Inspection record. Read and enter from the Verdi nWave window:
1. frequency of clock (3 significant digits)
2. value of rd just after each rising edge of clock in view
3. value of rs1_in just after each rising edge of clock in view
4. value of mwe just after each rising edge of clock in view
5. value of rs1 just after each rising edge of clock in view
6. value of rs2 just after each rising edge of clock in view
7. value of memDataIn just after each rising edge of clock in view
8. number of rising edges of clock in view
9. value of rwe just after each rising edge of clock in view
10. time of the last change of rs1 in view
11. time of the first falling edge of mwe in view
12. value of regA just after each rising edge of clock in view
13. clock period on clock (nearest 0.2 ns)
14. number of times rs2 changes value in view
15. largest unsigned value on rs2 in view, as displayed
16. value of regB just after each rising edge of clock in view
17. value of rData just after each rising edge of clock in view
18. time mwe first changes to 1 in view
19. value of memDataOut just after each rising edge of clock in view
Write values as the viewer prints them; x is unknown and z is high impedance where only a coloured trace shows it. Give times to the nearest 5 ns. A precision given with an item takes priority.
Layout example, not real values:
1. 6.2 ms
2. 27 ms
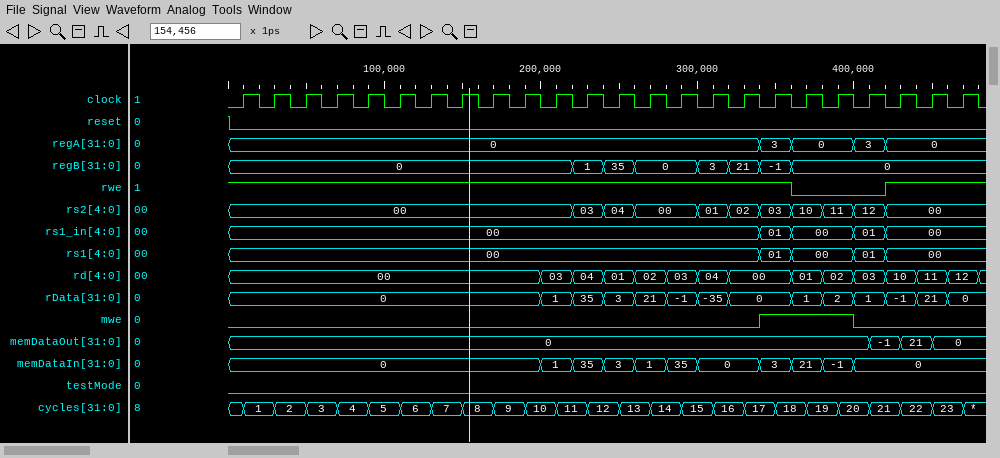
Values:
1. 50.0 MHz
2. 00, 00, 00, 00, 00, 00, 00, 00, 00, 00, 03, 04, 01, 02, 03, 04, 00, 00, 01, 02, 03, 10, 11, 12
3. 00, 00, 00, 00, 00, 00, 00, 00, 00, 00, 00, 00, 00, 00, 00, 00, 00, 01, 00, 00, 01, 00, 00, 00
4. 0 0 0 0 0 0 0 0 0 0 0 0 0 0 0 0 0 1 1 1 0 0 0 0
5. 00, 00, 00, 00, 00, 00, 00, 00, 00, 00, 00, 00, 00, 00, 00, 00, 00, 01, 00, 00, 01, 00, 00, 00
6. 00, 00, 00, 00, 00, 00, 00, 00, 00, 00, 00, 03, 04, 00, 00, 01, 02, 03, 10, 11, 12, 00, 00, 00
7. 0, 0, 0, 0, 0, 0, 0, 0, 0, 0, 1, 35, 3, 1, 35, 0, 0, 3, 21, -1, 0, 0, 0, 0
8. 24
9. 1 1 1 1 1 1 1 1 1 1 1 1 1 1 1 1 1 1 0 0 0 1 1 1
10. 420 ns
11. 400 ns
12. 0, 0, 0, 0, 0, 0, 0, 0, 0, 0, 0, 0, 0, 0, 0, 0, 0, 3, 0, 0, 3, 0, 0, 0
13. 20 ns
14. 10
15. 12
16. 0, 0, 0, 0, 0, 0, 0, 0, 0, 0, 0, 1, 35, 0, 0, 3, 21, -1, 0, 0, 0, 0, 0, 0
17. 0, 0, 0, 0, 0, 0, 0, 0, 0, 0, 1, 35, 3, 21, -1, -35, 0, 0, 1, 2, 1, -1, 21, 0
18. 340 ns
19. 0, 0, 0, 0, 0, 0, 0, 0, 0, 0, 0, 0, 0, 0, 0, 0, 0, 0, 0, 0, -1, 21, 0, 0
